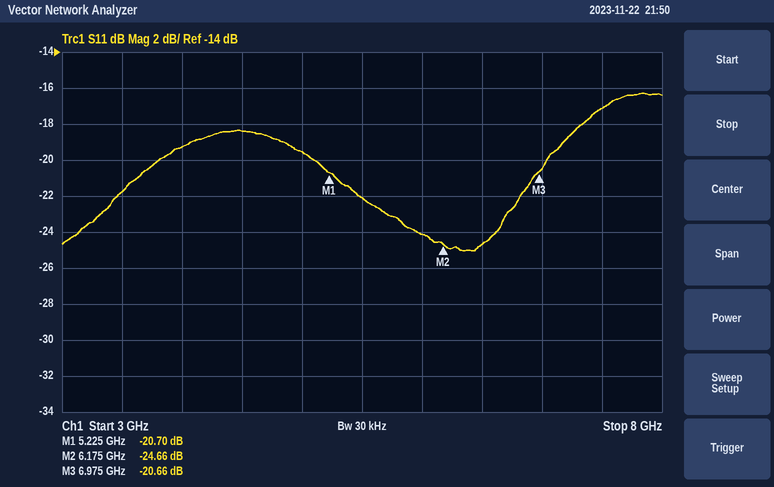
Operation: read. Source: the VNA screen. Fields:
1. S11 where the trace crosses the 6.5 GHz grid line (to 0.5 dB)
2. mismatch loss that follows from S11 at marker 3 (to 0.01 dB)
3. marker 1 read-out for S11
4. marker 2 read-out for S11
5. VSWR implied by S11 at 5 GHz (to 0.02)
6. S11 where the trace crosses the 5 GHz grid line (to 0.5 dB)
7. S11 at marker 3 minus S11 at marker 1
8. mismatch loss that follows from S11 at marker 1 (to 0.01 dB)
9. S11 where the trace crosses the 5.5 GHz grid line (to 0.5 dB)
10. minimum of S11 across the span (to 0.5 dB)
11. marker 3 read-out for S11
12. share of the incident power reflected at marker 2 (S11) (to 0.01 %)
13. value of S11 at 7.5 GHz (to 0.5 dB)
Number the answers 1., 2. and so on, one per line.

1. -24.5 dB
2. 0.04 dB
3. -20.70 dB
4. -24.66 dB
5. 1.24
6. -19.5 dB
7. 0.04 dB
8. 0.04 dB
9. -22.0 dB
10. -25.0 dB
11. -20.66 dB
12. 0.34 %
13. -17.0 dB
